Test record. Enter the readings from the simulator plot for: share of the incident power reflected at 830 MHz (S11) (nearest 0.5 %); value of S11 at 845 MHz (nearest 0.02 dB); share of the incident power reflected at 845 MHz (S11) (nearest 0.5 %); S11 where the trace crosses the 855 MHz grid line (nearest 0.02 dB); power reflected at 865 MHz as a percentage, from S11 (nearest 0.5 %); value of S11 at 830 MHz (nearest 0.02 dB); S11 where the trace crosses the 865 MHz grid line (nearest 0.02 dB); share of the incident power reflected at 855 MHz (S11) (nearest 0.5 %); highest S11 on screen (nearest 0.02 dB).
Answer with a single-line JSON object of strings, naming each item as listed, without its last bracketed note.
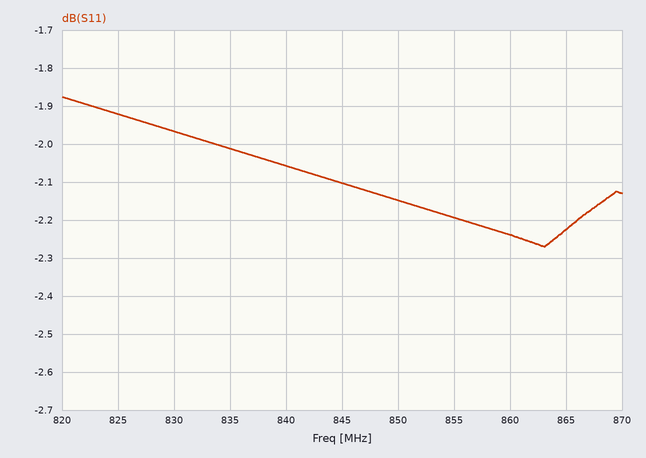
{"share of the incident power reflected at 830 MHz (S11)": "63.5 %", "value of S11 at 845 MHz": "-2.10 dB", "share of the incident power reflected at 845 MHz (S11)": "61.5 %", "S11 where the trace crosses the 855 MHz grid line": "-2.20 dB", "power reflected at 865 MHz as a percentage, from S11": "60.0 %", "value of S11 at 830 MHz": "-1.96 dB", "S11 where the trace crosses the 865 MHz grid line": "-2.22 dB", "share of the incident power reflected at 855 MHz (S11)": "60.5 %", "highest S11 on screen": "-1.88 dB"}
